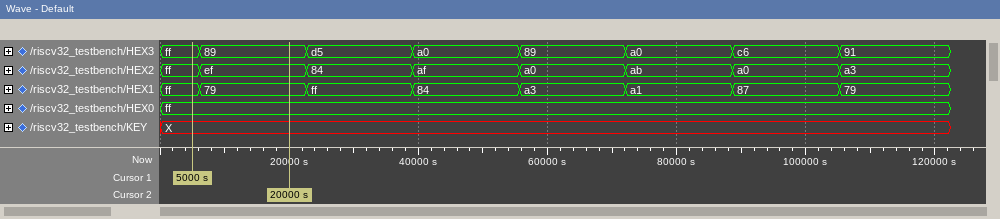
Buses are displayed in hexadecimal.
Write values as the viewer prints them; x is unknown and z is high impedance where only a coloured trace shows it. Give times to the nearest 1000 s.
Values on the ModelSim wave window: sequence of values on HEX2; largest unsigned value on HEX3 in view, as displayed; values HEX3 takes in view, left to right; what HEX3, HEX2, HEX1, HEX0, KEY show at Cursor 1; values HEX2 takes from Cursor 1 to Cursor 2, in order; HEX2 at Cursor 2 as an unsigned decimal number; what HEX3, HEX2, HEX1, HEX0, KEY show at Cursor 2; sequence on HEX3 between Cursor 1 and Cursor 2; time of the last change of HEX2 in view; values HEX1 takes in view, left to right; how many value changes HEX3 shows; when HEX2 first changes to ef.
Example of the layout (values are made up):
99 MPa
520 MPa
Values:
ff, ef, 84, af, a0, ab, a0, a3
ff
ff, 89, d5, a0, 89, a0, c6, 91
HEX3=ff, HEX2=ff, HEX1=ff, HEX0=ff, KEY=X
ff, ef
239
HEX3=89, HEX2=ef, HEX1=79, HEX0=ff, KEY=X
ff, 89
105000 s
ff, 79, ff, 84, a3, a1, 87, 79
7
6000 s
